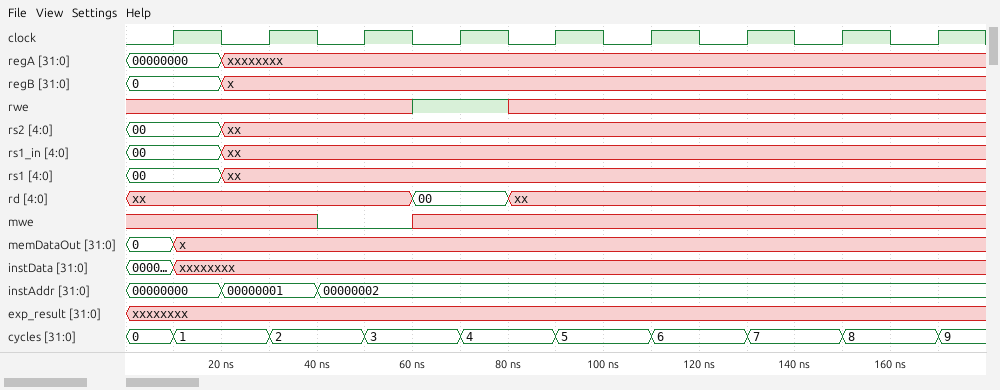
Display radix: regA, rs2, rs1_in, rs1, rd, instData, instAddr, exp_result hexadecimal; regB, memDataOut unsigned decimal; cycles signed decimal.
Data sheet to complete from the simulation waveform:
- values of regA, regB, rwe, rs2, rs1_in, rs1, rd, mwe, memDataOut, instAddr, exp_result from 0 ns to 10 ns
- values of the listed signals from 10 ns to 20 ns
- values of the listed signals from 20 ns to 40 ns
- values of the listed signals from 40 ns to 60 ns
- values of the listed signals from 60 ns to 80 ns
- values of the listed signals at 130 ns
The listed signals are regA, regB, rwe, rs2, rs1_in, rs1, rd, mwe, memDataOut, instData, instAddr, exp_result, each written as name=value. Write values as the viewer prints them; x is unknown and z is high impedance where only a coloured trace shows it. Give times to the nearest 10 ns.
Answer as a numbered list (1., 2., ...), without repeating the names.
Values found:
1. regA=00000000, regB=0, rwe=x, rs2=00, rs1_in=00, rs1=00, rd=xx, mwe=x, memDataOut=0, instAddr=00000000, exp_result=xxxxxxxx
2. regA=00000000, regB=0, rwe=x, rs2=00, rs1_in=00, rs1=00, rd=xx, mwe=x, memDataOut=x, instData=xxxxxxxx, instAddr=00000000, exp_result=xxxxxxxx
3. regA=xxxxxxxx, regB=x, rwe=x, rs2=xx, rs1_in=xx, rs1=xx, rd=xx, mwe=x, memDataOut=x, instData=xxxxxxxx, instAddr=00000001, exp_result=xxxxxxxx
4. regA=xxxxxxxx, regB=x, rwe=x, rs2=xx, rs1_in=xx, rs1=xx, rd=xx, mwe=0, memDataOut=x, instData=xxxxxxxx, instAddr=00000002, exp_result=xxxxxxxx
5. regA=xxxxxxxx, regB=x, rwe=1, rs2=xx, rs1_in=xx, rs1=xx, rd=00, mwe=x, memDataOut=x, instData=xxxxxxxx, instAddr=00000002, exp_result=xxxxxxxx
6. regA=xxxxxxxx, regB=x, rwe=x, rs2=xx, rs1_in=xx, rs1=xx, rd=xx, mwe=x, memDataOut=x, instData=xxxxxxxx, instAddr=00000002, exp_result=xxxxxxxx
